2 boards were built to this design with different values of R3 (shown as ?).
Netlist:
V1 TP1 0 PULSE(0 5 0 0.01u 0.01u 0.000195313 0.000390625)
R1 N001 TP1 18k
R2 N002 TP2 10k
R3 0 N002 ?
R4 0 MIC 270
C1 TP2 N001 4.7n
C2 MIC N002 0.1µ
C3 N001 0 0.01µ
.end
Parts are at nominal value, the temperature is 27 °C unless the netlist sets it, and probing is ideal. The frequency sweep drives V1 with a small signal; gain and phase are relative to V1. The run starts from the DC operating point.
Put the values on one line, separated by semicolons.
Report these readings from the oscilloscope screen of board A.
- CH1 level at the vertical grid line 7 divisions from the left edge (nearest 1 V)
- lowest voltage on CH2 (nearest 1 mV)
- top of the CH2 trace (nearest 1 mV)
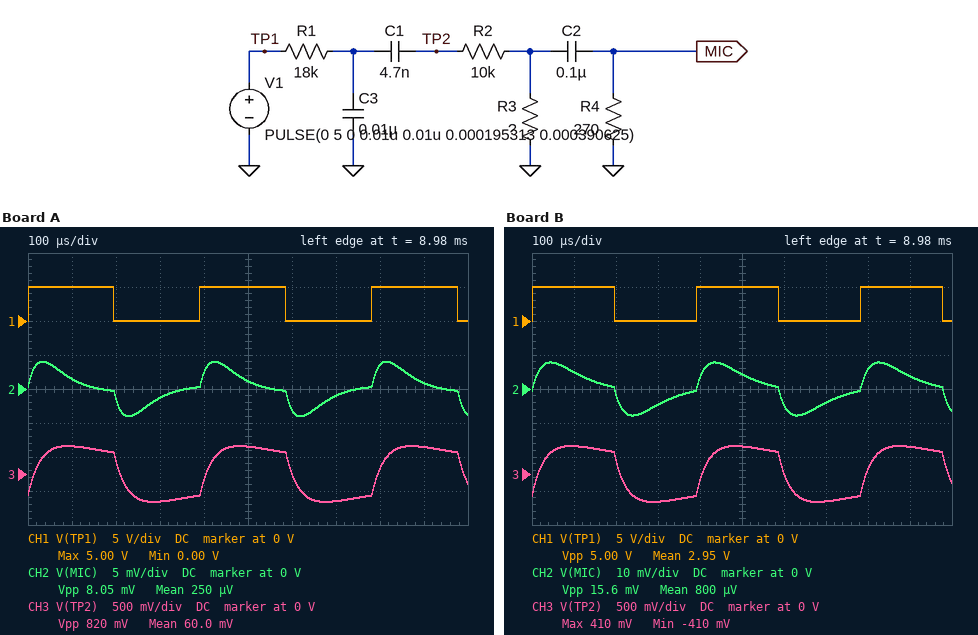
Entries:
0 V; -4 mV; 4 mV
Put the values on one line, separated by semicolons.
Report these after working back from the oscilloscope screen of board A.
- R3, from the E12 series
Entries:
180 Ω
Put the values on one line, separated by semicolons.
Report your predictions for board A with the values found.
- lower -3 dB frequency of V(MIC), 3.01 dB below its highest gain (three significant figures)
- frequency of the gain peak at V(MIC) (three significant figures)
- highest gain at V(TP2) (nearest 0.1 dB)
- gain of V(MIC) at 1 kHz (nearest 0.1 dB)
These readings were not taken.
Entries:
1.85 kHz; 4.38 kHz; -16.3 dB; -67.6 dB
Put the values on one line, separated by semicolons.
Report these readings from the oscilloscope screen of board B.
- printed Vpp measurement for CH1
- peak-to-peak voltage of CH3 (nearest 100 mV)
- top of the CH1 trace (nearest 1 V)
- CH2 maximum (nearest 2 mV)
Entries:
5.00 V; 800 mV; 5 V; 8 mV
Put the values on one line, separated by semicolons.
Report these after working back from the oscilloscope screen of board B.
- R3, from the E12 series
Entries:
560 Ω
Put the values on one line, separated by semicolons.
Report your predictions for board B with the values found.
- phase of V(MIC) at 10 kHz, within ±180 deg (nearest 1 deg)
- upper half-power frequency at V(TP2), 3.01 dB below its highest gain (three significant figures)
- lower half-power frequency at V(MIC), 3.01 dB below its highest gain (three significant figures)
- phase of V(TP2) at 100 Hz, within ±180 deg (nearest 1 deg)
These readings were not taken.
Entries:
-48 deg; 6.07 kHz; 1.33 kHz; 79 deg
